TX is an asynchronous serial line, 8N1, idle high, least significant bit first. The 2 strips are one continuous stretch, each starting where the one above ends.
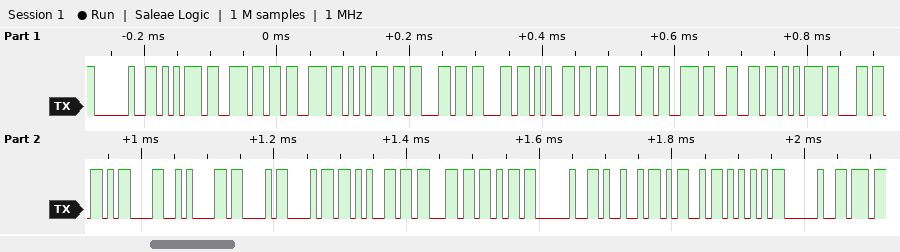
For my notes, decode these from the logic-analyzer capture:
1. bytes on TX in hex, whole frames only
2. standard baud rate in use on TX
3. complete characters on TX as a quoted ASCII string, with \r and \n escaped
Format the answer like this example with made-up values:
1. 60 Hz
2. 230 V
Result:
1. 20 75 6E 73 75 63 63 65 73 73 66 75 6C 0D 0A 43 68 65 63 6B 20 49 4D 55 20
2. 115200 baud
3. " unsuccessful\r\nCheck IMU "
